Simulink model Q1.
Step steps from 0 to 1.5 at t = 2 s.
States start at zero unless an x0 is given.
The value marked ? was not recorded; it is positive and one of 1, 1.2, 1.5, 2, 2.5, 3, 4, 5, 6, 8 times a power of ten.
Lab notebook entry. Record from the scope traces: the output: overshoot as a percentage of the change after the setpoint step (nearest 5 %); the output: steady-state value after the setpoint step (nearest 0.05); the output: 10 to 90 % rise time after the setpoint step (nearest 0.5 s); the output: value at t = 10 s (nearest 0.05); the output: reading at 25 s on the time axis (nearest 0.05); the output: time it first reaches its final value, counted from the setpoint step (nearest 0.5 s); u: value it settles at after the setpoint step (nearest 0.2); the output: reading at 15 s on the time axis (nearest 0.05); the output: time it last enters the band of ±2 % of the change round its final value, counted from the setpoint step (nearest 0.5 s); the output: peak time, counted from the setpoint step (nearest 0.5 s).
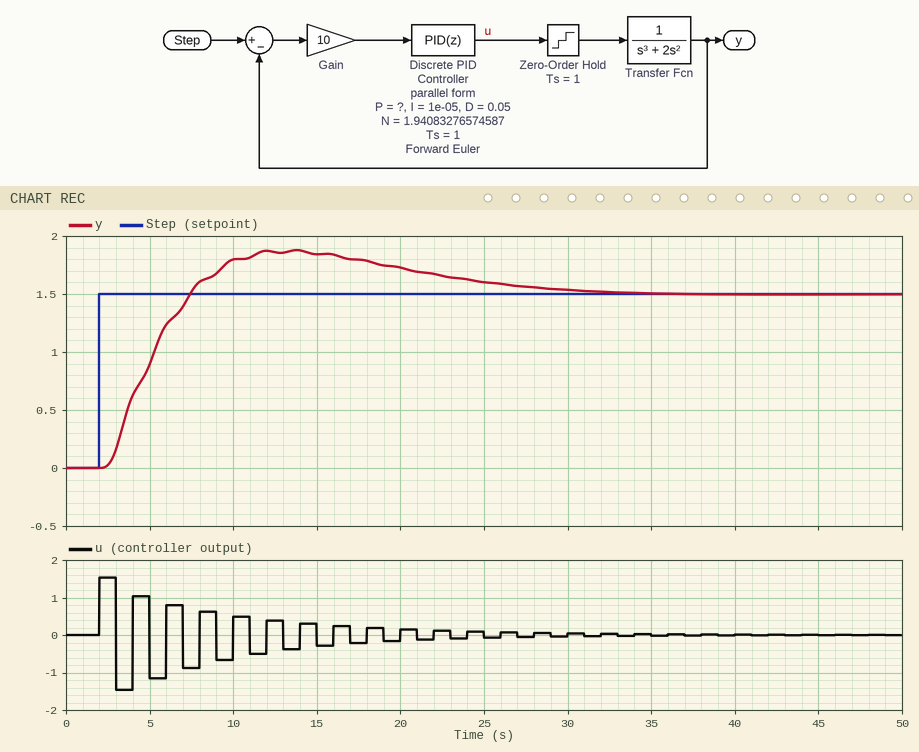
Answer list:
25 %
1.50
4.0 s
1.80
1.60
5.5 s
0.0
1.85
28.5 s
12.0 s
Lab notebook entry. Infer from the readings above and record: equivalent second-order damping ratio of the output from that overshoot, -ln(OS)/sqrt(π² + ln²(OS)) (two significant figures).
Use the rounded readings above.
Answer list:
0.40
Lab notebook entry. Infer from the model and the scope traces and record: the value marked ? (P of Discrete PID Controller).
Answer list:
0.005
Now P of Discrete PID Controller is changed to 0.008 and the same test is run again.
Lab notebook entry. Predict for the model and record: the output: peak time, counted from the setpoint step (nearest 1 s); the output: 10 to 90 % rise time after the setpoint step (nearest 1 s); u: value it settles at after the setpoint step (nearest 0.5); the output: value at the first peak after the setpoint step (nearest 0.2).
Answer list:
10 s
3 s
0.0
2.0
